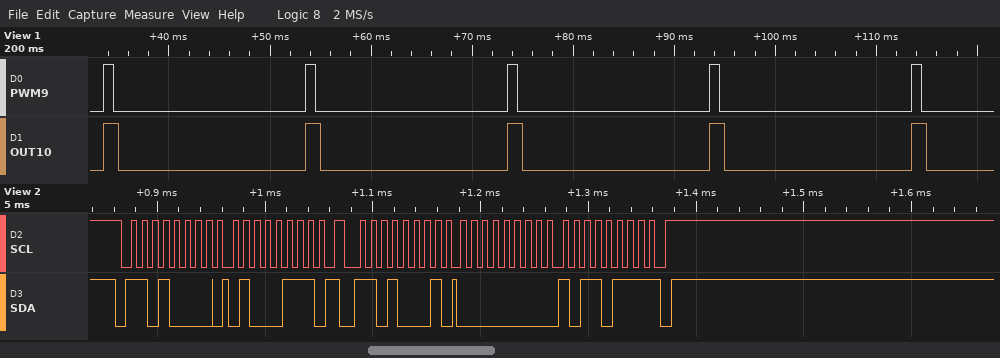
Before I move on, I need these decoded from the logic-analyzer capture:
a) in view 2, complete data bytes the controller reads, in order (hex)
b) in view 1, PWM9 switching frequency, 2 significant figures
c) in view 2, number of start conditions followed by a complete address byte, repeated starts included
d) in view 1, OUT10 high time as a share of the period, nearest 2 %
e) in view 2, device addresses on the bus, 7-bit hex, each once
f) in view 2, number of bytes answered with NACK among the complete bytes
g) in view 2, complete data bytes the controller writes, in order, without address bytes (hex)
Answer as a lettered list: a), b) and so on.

a) 00 B7
b) 50 Hz
c) 2
d) 8 %
e) 0x68
f) 1
g) 47
